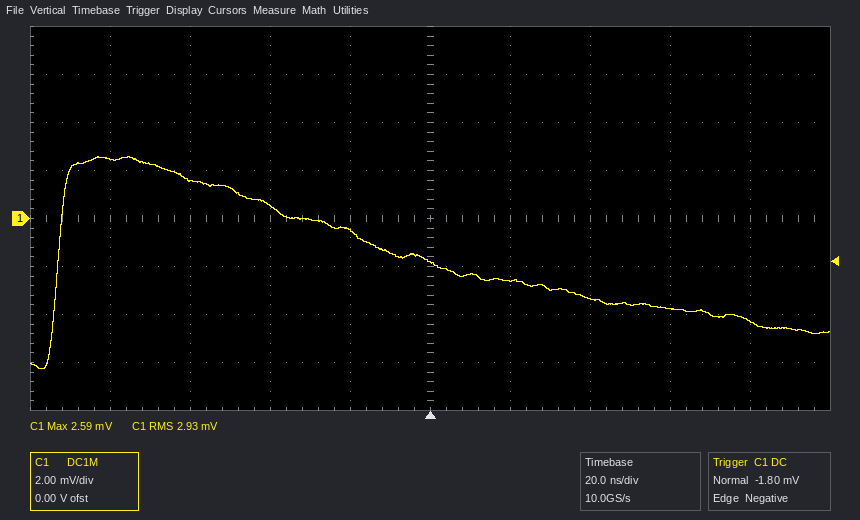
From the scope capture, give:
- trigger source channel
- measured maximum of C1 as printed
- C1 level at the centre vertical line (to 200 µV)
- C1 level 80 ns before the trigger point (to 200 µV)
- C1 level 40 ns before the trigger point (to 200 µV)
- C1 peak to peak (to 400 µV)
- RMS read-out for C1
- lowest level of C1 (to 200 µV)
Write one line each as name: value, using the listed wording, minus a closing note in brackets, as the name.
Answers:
trigger source channel: C1
measured maximum of C1 as printed: 2.59 mV
C1 level at the centre vertical line: -1.8 mV
C1 level 80 ns before the trigger point: 2.4 mV
C1 level 40 ns before the trigger point: 600 µV
C1 peak to peak: 8.8 mV
RMS read-out for C1: 2.93 mV
lowest level of C1: -6.2 mV
